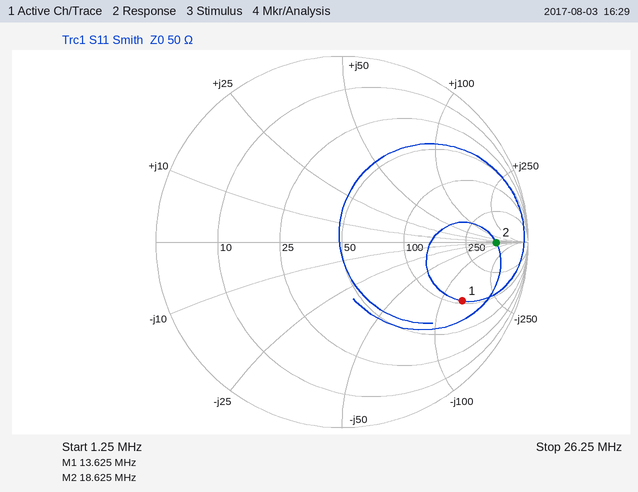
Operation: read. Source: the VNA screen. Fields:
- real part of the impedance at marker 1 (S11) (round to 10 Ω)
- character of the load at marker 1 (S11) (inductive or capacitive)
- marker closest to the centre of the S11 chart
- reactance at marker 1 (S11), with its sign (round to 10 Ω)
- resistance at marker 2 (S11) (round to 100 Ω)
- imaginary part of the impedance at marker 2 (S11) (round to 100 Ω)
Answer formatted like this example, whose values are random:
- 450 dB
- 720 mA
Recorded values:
- 110 Ω
- capacitive
- marker 1
- -140 Ω
- 500 Ω
- 0 Ω
